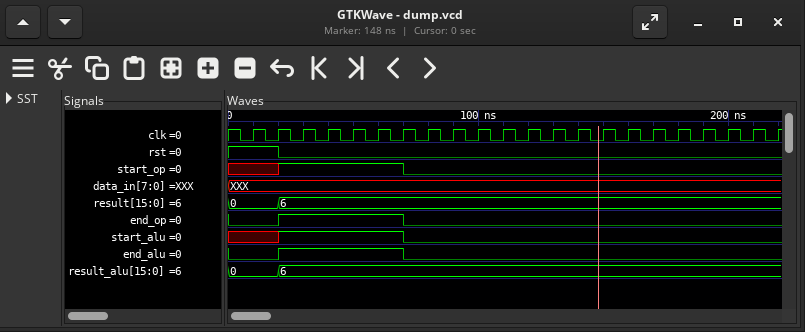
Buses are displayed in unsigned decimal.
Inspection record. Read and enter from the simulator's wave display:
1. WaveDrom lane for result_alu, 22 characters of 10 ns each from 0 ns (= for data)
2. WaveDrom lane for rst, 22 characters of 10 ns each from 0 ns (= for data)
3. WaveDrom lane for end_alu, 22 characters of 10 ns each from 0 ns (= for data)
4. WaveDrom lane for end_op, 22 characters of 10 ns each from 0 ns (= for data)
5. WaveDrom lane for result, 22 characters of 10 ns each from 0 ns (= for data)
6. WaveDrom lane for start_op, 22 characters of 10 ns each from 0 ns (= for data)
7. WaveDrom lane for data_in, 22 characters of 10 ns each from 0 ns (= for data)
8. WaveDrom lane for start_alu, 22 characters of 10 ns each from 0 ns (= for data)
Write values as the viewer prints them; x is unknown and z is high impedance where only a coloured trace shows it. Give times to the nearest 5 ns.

{name: 'result_alu', wave: '=.=...................', data: '0 6'}
{name: 'rst', wave: '1.0...................'}
{name: 'end_alu', wave: '0.1....0..............'}
{name: 'end_op', wave: '0.1....0..............'}
{name: 'result', wave: '=.=...................', data: '0 6'}
{name: 'start_op', wave: 'x.1....0..............'}
{name: 'data_in', wave: 'x.....................'}
{name: 'start_alu', wave: 'x.1....0..............'}
